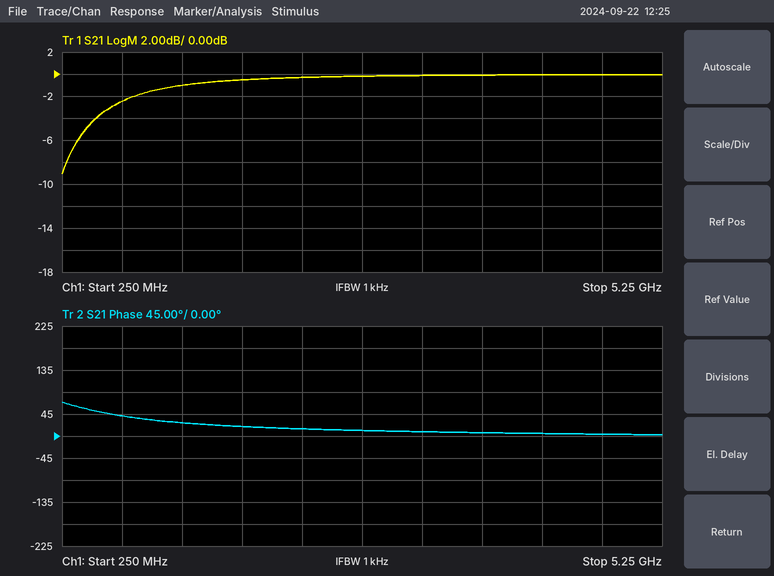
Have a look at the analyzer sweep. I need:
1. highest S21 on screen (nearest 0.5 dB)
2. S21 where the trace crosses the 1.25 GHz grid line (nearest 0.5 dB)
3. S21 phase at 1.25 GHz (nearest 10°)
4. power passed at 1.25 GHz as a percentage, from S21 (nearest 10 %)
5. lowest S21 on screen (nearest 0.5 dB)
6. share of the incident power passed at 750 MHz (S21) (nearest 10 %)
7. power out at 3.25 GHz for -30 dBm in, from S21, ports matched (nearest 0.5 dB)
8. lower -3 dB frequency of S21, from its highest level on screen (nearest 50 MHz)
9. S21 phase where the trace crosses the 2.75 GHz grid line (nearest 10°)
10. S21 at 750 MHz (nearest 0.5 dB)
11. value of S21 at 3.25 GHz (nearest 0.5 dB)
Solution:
0.0 dB
-1.0 dB
30°
80 %
-9.0 dB
60 %
-30.0 dBm
650 MHz
10°
-2.5 dB
0.0 dB
